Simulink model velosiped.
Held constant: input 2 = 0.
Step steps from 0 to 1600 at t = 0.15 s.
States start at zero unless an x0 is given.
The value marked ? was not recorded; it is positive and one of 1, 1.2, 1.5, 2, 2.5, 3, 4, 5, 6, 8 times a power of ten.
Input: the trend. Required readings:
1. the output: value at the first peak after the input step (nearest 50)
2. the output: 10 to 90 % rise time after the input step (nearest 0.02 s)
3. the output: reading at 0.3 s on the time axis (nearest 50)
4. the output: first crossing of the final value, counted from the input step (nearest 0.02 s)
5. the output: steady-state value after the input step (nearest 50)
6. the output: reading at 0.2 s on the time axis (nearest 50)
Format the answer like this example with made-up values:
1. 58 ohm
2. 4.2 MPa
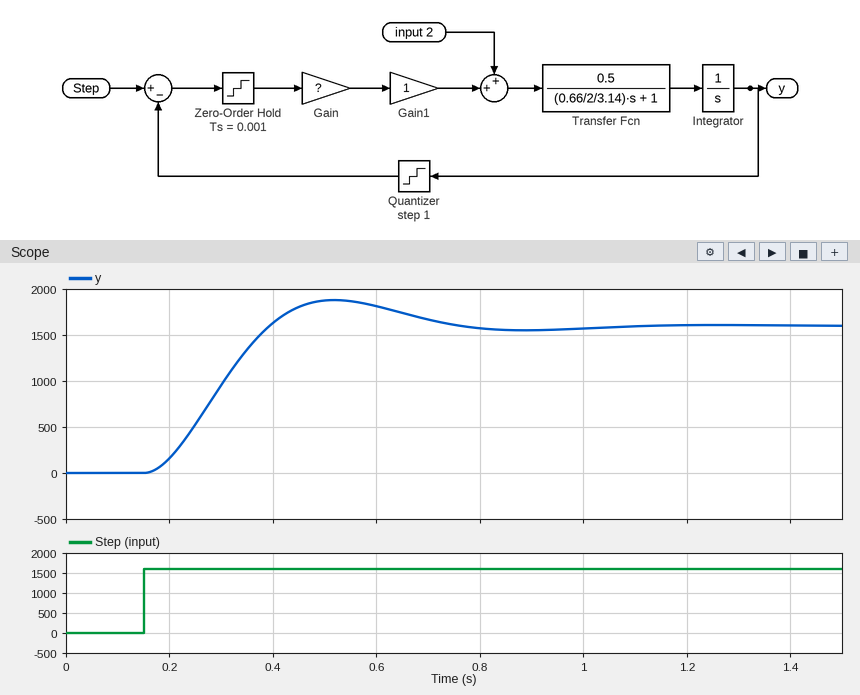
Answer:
1. 1900
2. 0.16 s
3. 950
4. 0.24 s
5. 1600
6. 150
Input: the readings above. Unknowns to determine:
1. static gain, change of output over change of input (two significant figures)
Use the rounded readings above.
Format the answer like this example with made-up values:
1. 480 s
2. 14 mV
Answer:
1. 1.0
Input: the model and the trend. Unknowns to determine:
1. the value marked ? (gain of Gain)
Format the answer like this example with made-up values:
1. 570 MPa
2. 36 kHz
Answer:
1. 20
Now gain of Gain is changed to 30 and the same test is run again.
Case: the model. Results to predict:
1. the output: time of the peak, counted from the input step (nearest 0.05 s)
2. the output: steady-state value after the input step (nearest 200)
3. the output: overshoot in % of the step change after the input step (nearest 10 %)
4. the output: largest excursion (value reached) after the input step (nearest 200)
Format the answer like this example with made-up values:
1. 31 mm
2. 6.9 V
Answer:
1. 0.30 s
2. 1600
3. 30 %
4. 2000
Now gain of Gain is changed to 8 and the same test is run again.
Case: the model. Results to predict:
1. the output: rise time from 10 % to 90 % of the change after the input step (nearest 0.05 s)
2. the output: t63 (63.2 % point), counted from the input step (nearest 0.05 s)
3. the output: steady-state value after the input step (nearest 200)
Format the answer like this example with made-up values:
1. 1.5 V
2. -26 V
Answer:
1. 0.40 s
2. 0.30 s
3. 1600
